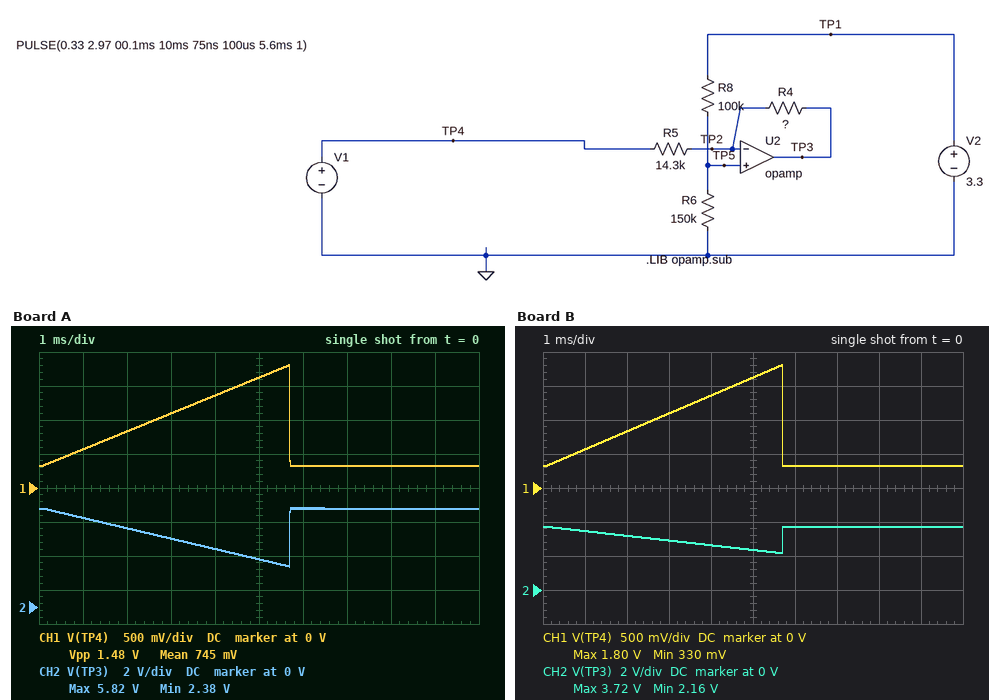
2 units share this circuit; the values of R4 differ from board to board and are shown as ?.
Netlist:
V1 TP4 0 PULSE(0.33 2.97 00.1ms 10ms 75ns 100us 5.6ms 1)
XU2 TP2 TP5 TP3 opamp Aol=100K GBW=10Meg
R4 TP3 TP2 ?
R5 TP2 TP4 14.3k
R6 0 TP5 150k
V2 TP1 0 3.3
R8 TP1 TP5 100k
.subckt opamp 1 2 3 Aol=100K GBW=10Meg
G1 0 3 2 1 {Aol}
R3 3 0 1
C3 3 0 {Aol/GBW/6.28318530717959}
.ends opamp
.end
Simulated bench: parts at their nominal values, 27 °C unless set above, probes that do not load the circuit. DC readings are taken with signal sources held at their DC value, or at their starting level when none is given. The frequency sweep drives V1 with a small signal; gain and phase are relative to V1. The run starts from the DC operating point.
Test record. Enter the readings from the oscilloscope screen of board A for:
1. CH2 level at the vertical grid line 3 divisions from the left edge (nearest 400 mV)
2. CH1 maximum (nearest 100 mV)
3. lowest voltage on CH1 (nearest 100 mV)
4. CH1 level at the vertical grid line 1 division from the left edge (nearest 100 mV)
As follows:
4.0 V
1.8 V
300 mV
600 mV
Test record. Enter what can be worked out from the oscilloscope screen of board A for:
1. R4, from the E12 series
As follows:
33 kΩ
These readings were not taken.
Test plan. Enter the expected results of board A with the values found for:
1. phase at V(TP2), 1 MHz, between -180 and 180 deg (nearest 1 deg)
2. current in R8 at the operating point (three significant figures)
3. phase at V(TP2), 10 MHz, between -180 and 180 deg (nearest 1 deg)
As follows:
72 deg
13.2 µA
17 deg
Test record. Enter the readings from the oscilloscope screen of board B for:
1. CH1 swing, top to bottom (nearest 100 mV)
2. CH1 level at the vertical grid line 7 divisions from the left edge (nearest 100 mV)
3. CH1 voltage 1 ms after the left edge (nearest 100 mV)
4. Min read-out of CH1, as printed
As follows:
1.5 V
300 mV
600 mV
330 mV
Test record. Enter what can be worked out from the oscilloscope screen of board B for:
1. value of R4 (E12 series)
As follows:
15 kΩ
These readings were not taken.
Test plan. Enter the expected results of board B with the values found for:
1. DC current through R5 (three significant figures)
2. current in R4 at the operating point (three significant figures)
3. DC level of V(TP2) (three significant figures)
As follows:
115 µA
115 µA
1.98 V
